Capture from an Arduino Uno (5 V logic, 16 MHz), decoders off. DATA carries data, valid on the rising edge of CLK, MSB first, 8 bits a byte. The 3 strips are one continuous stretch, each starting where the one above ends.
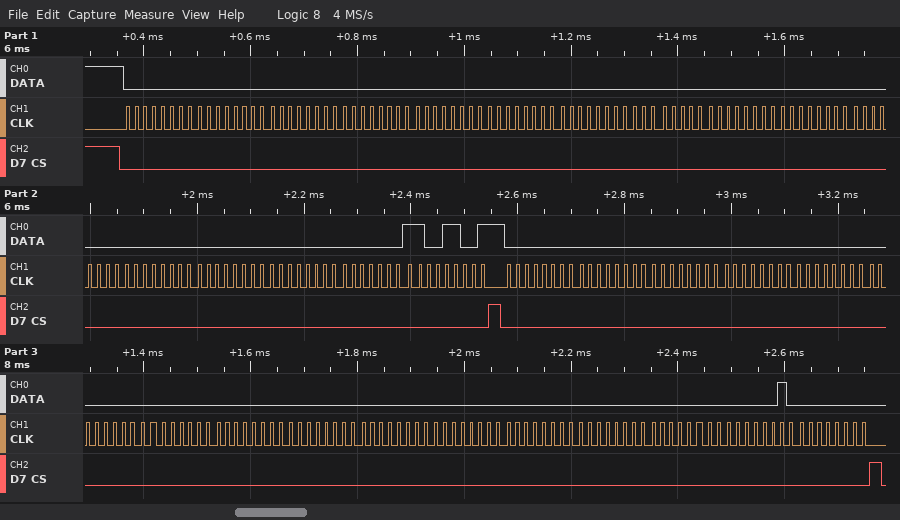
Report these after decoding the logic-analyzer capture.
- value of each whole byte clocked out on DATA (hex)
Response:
0x00 0x00 0x00 0x00 0x00 0x00 0x00 0x00 0x00 0x00 0x00 0x00 0x00 0x00 0x01 0x99 0x00 0x00 0x00 0x00 0x00 0x00 0x00 0x00 0x00 0x00 0x00 0x00 0x00 0x00 0x02 0x00
